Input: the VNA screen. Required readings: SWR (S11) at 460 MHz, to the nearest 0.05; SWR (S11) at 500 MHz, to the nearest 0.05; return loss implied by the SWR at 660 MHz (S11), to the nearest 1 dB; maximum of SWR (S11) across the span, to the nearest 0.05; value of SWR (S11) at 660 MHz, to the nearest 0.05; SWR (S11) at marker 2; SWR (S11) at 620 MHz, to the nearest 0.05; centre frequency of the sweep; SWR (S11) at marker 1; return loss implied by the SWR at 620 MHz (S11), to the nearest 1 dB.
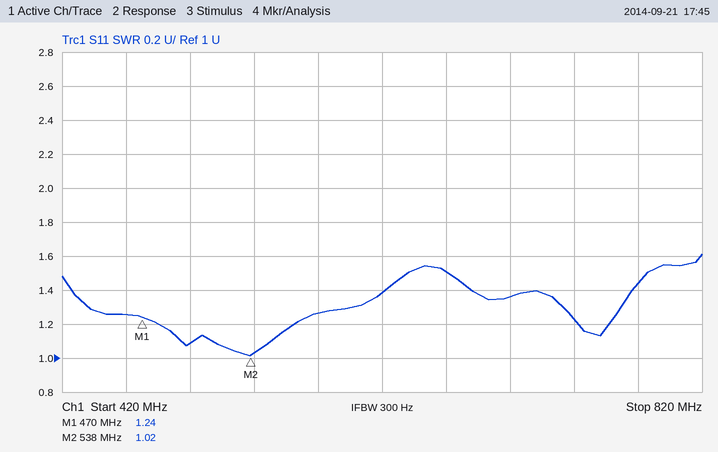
1.25
1.10
14 dB
1.60
1.50
1.02
1.40
620 MHz
1.24
16 dB
